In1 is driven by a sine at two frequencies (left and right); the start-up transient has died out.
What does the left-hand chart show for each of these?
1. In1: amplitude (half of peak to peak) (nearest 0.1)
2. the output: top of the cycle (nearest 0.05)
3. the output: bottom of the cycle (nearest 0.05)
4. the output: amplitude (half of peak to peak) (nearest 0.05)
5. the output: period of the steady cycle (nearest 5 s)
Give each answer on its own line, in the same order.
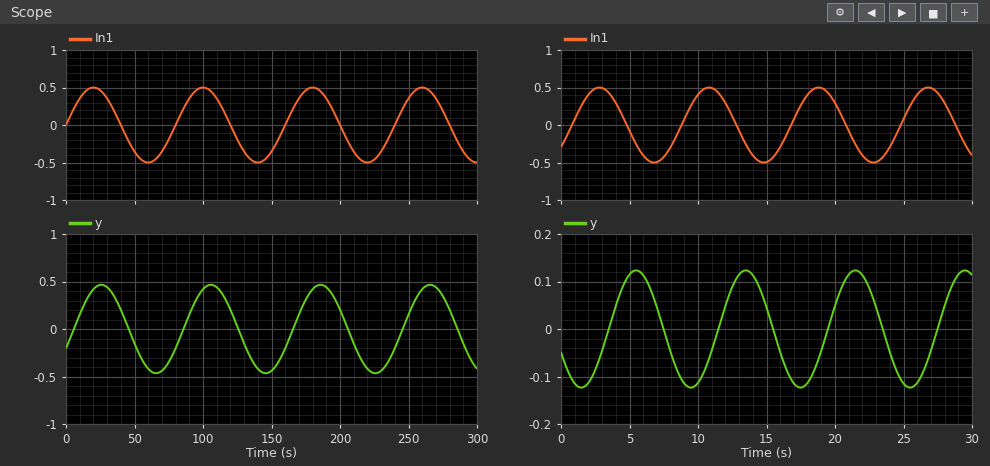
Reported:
0.5
0.45
-0.45
0.45
80 s
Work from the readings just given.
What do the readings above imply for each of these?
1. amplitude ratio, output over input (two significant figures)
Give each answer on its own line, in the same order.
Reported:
0.90
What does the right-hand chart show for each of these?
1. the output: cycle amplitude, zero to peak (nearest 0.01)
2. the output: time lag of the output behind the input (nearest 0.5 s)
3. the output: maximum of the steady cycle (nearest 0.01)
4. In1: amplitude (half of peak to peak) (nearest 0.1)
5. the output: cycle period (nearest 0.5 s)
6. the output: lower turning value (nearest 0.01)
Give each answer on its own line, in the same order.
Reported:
0.12
2.5 s
0.12
0.5
8.0 s
-0.12
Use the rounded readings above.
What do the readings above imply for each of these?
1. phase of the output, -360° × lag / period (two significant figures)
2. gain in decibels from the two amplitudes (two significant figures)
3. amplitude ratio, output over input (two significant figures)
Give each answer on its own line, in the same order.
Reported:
-110°
-12 dB
0.24
